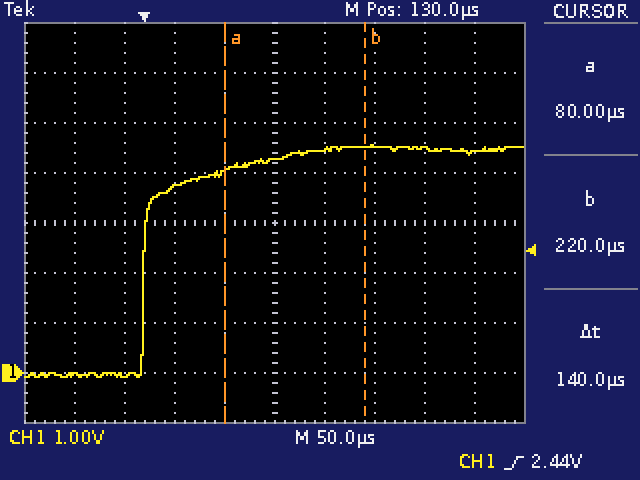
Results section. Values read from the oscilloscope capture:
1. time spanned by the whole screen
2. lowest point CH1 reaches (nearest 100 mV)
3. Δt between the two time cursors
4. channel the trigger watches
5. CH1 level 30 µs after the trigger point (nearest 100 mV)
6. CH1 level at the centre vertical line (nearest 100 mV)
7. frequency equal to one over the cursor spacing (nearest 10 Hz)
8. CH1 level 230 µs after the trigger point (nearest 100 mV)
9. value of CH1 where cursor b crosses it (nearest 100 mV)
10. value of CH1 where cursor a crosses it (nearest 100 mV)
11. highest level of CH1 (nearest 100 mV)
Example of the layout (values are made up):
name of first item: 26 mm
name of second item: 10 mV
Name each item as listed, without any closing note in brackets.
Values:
time spanned by the whole screen: 500 µs
lowest point CH1 reaches: -100 mV
Δt between the two time cursors: 140 µs
channel the trigger watches: CH1
CH1 level 30 µs after the trigger point: 3.7 V
CH1 level at the centre vertical line: 4.3 V
frequency equal to one over the cursor spacing: 7.14 kHz
CH1 level 230 µs after the trigger point: 4.5 V
value of CH1 where cursor b crosses it: 4.5 V
value of CH1 where cursor a crosses it: 4.0 V
highest level of CH1: 4.6 V
